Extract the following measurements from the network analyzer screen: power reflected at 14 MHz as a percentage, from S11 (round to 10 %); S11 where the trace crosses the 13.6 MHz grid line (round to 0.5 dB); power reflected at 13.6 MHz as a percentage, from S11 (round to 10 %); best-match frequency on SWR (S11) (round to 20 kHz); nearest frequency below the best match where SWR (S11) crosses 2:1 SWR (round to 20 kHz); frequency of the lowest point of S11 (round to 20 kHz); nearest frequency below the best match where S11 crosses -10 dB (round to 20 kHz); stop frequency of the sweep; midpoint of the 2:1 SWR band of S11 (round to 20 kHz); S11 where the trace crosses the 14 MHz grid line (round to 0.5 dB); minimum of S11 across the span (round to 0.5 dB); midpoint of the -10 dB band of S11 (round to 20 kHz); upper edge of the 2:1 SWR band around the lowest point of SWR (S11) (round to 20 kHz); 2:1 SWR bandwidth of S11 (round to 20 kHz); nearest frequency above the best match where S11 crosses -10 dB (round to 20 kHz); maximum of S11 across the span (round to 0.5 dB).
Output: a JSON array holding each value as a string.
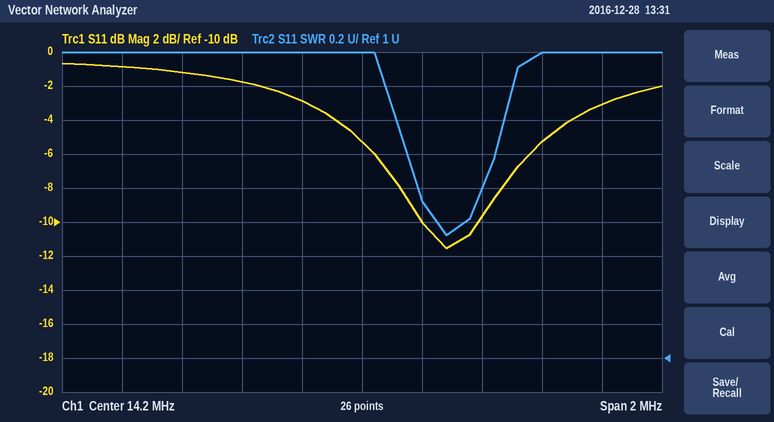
["50 %", "-1.0 dB", "80 %", "14.48 MHz", "14.38 MHz", "14.48 MHz", "14.40 MHz", "15.2 MHz", "14.50 MHz", "-3.0 dB", "-11.5 dB", "14.50 MHz", "14.60 MHz", "220 kHz", "14.58 MHz", "-0.5 dB"]
